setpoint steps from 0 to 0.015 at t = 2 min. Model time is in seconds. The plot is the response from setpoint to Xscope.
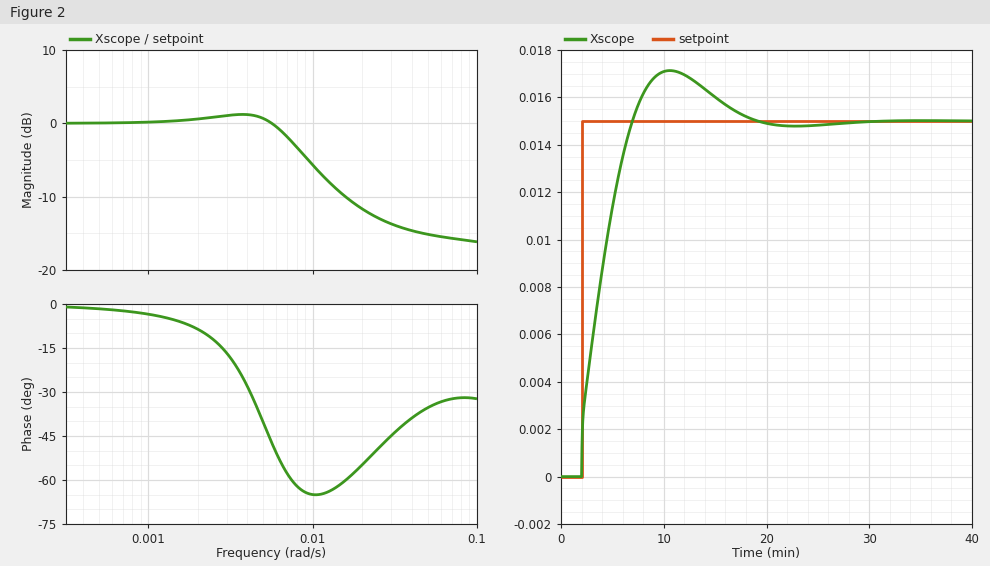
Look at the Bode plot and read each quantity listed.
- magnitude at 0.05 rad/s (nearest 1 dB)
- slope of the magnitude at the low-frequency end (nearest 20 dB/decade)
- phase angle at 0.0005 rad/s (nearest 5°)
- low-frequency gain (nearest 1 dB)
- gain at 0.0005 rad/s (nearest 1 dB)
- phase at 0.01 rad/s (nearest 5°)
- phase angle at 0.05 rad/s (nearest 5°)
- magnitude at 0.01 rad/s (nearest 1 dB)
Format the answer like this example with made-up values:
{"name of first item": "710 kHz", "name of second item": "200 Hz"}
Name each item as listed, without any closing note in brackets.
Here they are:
{"magnitude at 0.05 rad/s": "-15 dB", "slope of the magnitude at the low-frequency end": "0 dB/decade", "phase angle at 0.0005 rad/s": "0°", "low-frequency gain": "0 dB", "gain at 0.0005 rad/s": "0 dB", "phase at 0.01 rad/s": "-65°", "phase angle at 0.05 rad/s": "-35°", "magnitude at 0.01 rad/s": "-6 dB"}
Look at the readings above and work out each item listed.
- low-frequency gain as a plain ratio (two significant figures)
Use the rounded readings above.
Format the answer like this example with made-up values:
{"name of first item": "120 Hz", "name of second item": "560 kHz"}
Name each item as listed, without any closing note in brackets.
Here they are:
{"low-frequency gain as a plain ratio": "1.0"}
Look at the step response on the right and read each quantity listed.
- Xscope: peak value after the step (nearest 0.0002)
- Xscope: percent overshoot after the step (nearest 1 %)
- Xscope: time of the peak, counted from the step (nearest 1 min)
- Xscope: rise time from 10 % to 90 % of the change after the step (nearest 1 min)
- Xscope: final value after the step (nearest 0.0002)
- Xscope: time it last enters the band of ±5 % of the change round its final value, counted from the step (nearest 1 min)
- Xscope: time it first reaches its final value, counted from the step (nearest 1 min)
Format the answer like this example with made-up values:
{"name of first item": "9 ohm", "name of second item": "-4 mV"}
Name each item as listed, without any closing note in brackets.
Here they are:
{"Xscope: peak value after the step": "0.0172", "Xscope: percent overshoot after the step": "14 %", "Xscope: time of the peak, counted from the step": "9 min", "Xscope: rise time from 10 % to 90 % of the change after the step": "4 min", "Xscope: final value after the step": "0.0150", "Xscope: time it last enters the band of ±5 % of the change round its final value, counted from the step": "14 min", "Xscope: time it first reaches its final value, counted from the step": "5 min"}
